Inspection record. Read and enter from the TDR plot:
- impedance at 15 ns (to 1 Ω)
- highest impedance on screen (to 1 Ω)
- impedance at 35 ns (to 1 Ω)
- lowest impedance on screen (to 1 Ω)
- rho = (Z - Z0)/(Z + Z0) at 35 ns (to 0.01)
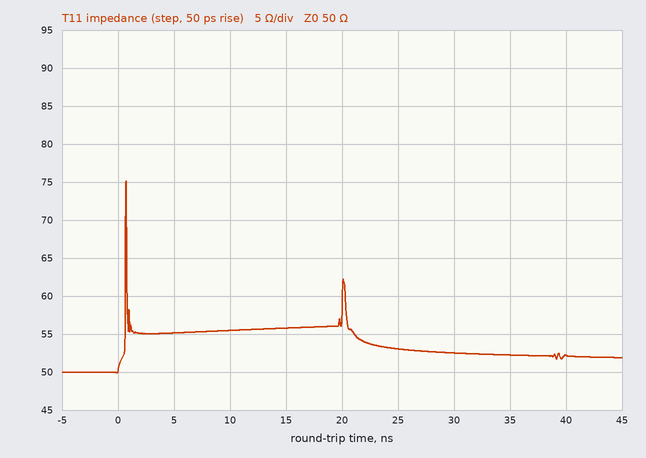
56 Ω
75 Ω
52 Ω
50 Ω
+0.02
